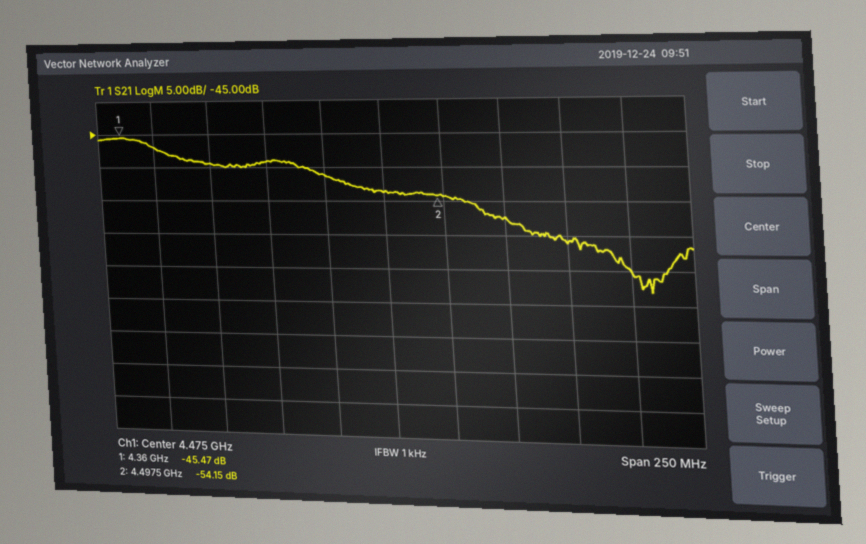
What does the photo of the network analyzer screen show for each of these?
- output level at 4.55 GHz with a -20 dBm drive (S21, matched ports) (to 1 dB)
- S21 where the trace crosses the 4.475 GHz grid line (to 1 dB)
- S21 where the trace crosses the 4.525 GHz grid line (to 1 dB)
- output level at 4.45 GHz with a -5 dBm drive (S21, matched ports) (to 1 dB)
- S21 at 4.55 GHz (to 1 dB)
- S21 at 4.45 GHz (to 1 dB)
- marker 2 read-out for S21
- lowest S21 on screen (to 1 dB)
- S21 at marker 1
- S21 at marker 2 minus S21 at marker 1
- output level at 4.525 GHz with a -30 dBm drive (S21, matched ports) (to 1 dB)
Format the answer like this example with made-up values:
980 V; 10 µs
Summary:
-81 dBm; -54 dB; -57 dB; -56 dBm; -61 dB; -51 dB; -54.15 dB; -68 dB; -45.47 dB; -8.68 dB; -87 dBm
